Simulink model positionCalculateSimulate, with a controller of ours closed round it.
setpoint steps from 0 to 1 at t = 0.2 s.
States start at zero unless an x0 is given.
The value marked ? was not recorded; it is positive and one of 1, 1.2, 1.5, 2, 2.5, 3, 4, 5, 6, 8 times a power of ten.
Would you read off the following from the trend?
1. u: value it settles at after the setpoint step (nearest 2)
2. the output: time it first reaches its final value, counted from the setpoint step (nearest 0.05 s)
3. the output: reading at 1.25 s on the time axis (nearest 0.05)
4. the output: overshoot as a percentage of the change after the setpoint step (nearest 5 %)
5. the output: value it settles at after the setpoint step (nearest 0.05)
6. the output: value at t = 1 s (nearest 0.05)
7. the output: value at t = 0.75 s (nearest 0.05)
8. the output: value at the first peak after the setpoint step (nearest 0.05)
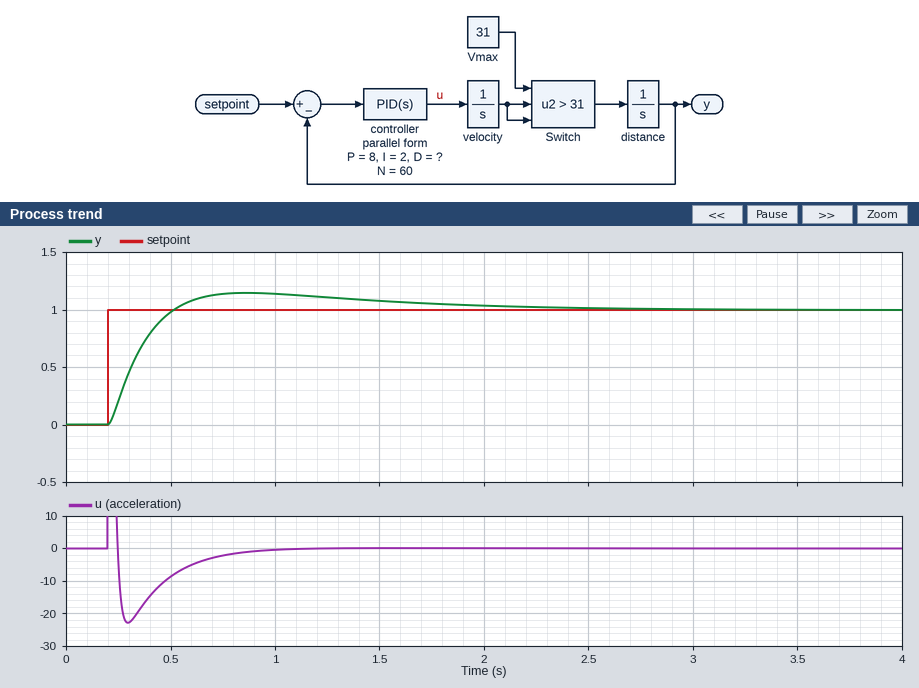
0
0.30 s
1.10
15 %
1.00
1.15
1.15
1.15
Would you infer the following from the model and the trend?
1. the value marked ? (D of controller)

6
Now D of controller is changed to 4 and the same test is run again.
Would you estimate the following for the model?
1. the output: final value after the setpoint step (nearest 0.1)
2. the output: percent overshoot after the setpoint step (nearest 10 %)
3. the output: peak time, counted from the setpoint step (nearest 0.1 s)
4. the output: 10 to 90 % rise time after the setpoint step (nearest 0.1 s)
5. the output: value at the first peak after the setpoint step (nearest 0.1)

1.0
20 %
0.8 s
0.3 s
1.2
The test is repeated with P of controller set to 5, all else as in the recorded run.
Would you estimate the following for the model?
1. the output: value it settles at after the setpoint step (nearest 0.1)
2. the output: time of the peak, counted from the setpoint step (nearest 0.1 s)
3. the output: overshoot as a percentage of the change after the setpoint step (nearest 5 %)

1.0
0.8 s
10 %
